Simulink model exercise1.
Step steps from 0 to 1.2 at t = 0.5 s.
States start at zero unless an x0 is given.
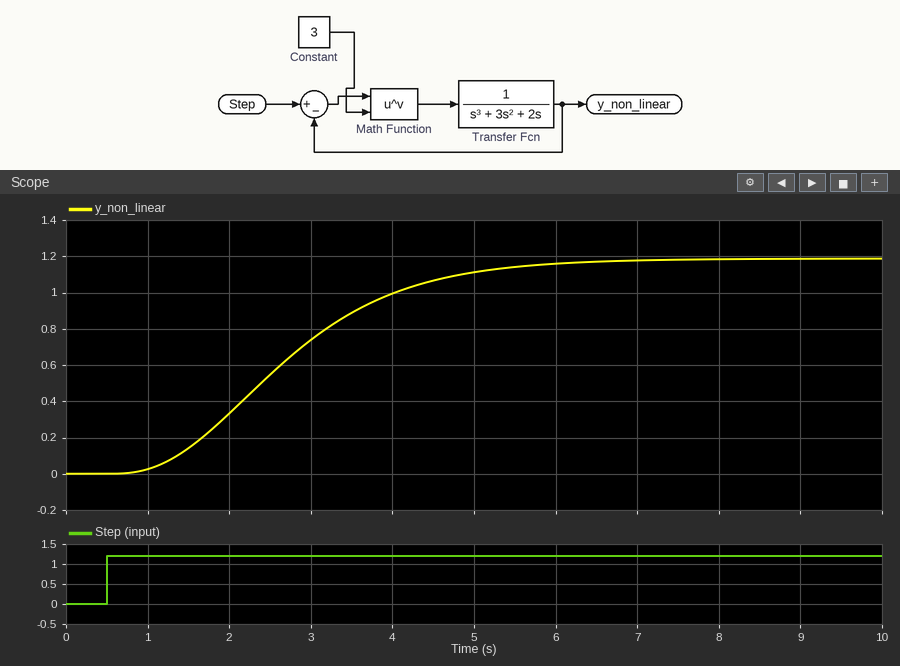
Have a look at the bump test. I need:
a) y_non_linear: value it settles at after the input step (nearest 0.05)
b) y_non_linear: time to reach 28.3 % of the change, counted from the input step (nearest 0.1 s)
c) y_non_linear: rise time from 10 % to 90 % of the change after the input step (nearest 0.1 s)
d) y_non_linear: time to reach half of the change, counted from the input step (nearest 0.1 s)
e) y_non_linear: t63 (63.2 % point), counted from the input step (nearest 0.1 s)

1.20
1.5 s
3.1 s
2.1 s
2.5 s
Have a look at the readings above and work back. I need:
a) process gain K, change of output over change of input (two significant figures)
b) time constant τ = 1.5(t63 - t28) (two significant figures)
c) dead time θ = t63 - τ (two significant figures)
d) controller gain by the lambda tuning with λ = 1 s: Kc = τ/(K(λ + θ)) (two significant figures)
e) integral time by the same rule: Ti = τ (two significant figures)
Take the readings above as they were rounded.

1.0
1.5 s
1.0 s
0.75
1.5 s
